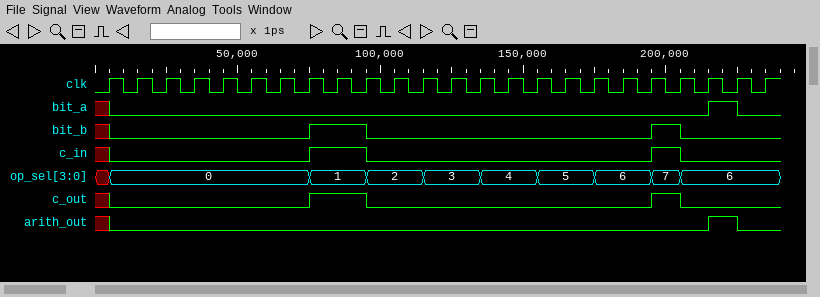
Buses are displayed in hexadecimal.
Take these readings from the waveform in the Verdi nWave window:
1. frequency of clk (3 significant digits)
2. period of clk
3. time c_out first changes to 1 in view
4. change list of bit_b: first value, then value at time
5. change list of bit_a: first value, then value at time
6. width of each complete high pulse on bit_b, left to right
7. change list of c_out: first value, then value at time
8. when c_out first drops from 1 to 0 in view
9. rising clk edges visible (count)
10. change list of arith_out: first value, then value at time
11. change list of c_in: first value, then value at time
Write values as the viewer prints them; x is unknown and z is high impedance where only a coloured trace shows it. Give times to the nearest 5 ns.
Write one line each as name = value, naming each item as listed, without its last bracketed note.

frequency of clk = 100 MHz
period of clk = 10 ns
time c_out first changes to 1 in view = 75 ns
change list of bit_b: first value, then value at time = x, 0 at 5 ns, 1 at 75 ns, 0 at 95 ns, 1 at 195 ns, 0 at 205 ns
change list of bit_a: first value, then value at time = x, 0 at 5 ns, 1 at 215 ns, 0 at 225 ns
width of each complete high pulse on bit_b, left to right = 20 ns, 10 ns
change list of c_out: first value, then value at time = x, 0 at 5 ns, 1 at 75 ns, 0 at 95 ns, 1 at 195 ns, 0 at 205 ns
when c_out first drops from 1 to 0 in view = 95 ns
rising clk edges visible = 24
change list of arith_out: first value, then value at time = x, 0 at 5 ns, 1 at 215 ns, 0 at 225 ns
change list of c_in: first value, then value at time = x, 0 at 5 ns, 1 at 75 ns, 0 at 95 ns, 1 at 195 ns, 0 at 205 ns
